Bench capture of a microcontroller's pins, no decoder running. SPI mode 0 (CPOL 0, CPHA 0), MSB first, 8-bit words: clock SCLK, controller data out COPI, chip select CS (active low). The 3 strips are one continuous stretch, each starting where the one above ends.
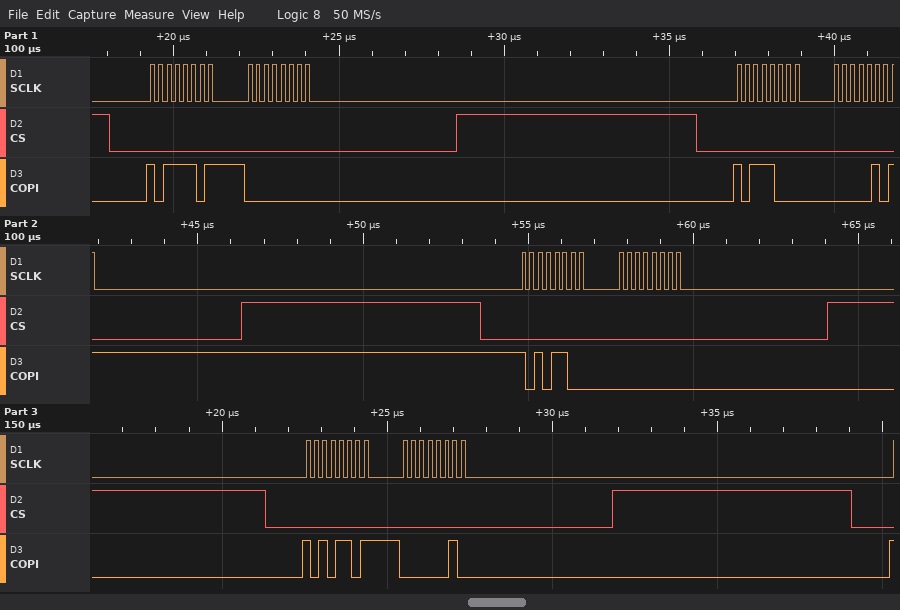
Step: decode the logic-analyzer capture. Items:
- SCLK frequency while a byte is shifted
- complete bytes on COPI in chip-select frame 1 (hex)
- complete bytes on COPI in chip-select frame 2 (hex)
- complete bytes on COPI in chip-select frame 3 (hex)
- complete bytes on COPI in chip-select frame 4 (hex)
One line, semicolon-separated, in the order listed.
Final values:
4 MHz; BD 00; B8 05; AC 00; AD 02
